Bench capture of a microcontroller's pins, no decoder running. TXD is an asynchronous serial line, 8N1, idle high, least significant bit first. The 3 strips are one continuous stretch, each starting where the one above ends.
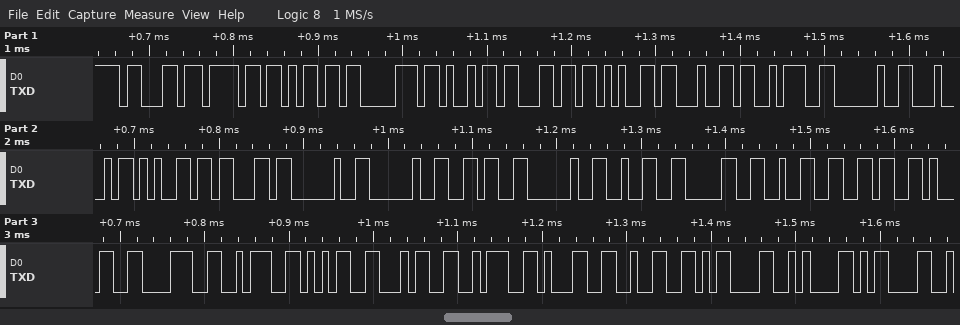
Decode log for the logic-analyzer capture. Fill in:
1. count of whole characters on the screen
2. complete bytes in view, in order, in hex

32
63 6F 6D 70 69 6C 65 64 3A 20 44 65 63 20 20 36 20 32 30 32 36 31 38 3A 35 34 3A 31 32 0D 0A 0D
